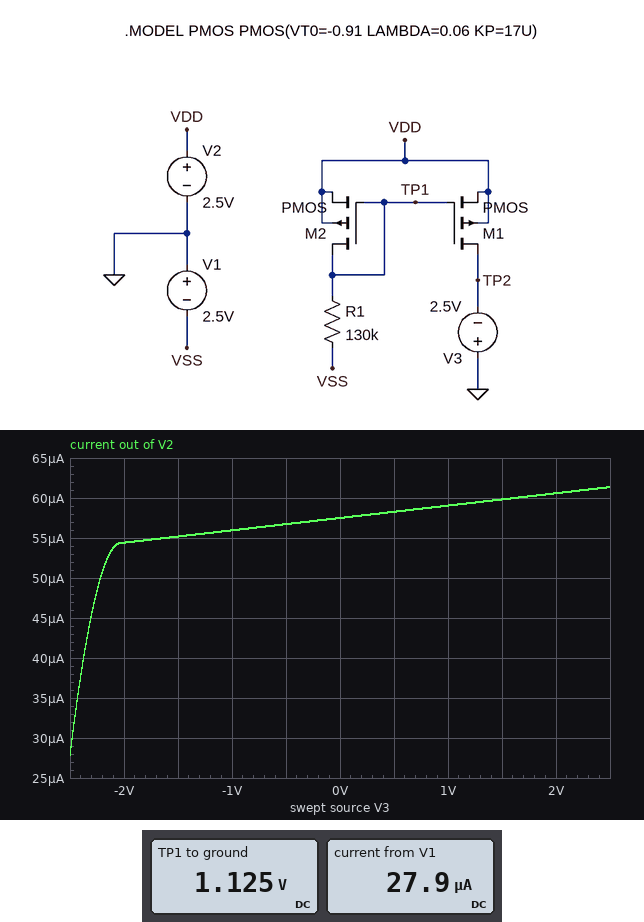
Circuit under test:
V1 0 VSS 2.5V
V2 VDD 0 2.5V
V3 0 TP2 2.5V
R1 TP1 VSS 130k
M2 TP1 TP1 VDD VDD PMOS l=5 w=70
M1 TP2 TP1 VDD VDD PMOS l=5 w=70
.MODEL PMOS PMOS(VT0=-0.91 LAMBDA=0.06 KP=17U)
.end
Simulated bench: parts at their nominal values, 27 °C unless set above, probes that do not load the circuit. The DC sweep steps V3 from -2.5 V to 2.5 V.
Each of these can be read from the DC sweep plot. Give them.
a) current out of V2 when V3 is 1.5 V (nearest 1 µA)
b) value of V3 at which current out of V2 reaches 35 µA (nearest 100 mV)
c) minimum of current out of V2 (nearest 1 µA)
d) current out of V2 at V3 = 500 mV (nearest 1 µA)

60 µA
-2.4 V
28 µA
58 µA
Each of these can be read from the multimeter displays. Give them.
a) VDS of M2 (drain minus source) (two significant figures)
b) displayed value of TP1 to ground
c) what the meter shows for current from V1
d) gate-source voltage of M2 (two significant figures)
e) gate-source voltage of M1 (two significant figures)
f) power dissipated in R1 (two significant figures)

-1.4 V
1.125 V
27.9 µA
-1.4 V
-1.4 V
100 µW
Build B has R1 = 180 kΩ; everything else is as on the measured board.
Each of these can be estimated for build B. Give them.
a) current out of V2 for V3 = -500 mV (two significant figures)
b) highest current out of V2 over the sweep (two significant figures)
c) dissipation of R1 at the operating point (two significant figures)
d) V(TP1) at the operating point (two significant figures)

42 µA
45 µA
76 µW
1.2 V
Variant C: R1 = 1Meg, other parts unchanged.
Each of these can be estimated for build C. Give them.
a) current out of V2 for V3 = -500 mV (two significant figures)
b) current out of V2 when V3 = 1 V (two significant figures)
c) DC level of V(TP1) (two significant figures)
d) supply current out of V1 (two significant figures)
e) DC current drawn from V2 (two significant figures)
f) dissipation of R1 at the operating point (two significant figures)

8.0 µA
8.4 µA
1.4 V
3.9 µA
8.7 µA
15 µW
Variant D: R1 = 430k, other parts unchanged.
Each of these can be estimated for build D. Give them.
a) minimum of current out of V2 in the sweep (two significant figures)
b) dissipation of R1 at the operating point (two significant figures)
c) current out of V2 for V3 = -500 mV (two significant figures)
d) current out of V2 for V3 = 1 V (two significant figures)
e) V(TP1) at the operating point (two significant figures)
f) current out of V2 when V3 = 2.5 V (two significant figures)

8.9 µA
34 µW
18 µA
19 µA
1.3 V
20 µA
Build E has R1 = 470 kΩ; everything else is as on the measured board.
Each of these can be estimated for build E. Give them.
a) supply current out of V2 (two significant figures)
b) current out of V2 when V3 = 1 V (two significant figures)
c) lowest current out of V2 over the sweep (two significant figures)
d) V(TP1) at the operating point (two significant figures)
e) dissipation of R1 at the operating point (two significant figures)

18 µA
17 µA
8.2 µA
1.3 V
31 µW
